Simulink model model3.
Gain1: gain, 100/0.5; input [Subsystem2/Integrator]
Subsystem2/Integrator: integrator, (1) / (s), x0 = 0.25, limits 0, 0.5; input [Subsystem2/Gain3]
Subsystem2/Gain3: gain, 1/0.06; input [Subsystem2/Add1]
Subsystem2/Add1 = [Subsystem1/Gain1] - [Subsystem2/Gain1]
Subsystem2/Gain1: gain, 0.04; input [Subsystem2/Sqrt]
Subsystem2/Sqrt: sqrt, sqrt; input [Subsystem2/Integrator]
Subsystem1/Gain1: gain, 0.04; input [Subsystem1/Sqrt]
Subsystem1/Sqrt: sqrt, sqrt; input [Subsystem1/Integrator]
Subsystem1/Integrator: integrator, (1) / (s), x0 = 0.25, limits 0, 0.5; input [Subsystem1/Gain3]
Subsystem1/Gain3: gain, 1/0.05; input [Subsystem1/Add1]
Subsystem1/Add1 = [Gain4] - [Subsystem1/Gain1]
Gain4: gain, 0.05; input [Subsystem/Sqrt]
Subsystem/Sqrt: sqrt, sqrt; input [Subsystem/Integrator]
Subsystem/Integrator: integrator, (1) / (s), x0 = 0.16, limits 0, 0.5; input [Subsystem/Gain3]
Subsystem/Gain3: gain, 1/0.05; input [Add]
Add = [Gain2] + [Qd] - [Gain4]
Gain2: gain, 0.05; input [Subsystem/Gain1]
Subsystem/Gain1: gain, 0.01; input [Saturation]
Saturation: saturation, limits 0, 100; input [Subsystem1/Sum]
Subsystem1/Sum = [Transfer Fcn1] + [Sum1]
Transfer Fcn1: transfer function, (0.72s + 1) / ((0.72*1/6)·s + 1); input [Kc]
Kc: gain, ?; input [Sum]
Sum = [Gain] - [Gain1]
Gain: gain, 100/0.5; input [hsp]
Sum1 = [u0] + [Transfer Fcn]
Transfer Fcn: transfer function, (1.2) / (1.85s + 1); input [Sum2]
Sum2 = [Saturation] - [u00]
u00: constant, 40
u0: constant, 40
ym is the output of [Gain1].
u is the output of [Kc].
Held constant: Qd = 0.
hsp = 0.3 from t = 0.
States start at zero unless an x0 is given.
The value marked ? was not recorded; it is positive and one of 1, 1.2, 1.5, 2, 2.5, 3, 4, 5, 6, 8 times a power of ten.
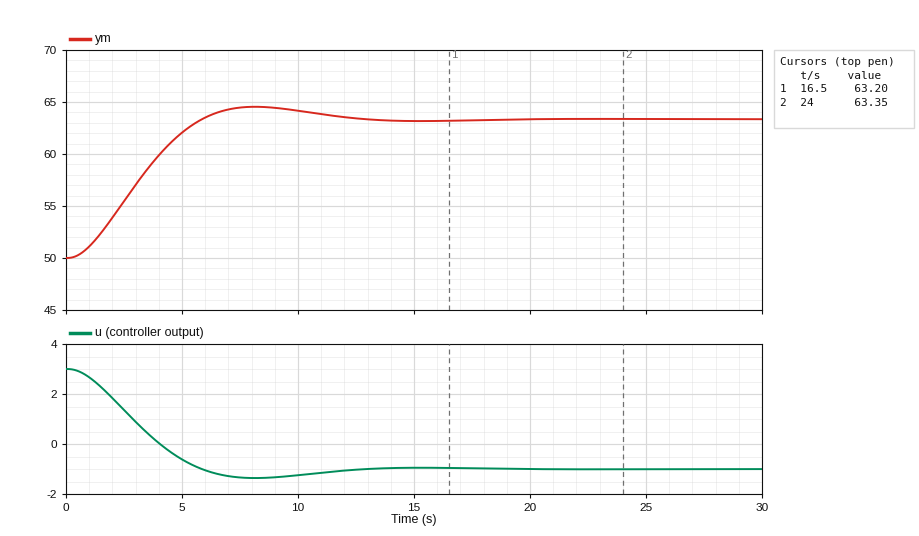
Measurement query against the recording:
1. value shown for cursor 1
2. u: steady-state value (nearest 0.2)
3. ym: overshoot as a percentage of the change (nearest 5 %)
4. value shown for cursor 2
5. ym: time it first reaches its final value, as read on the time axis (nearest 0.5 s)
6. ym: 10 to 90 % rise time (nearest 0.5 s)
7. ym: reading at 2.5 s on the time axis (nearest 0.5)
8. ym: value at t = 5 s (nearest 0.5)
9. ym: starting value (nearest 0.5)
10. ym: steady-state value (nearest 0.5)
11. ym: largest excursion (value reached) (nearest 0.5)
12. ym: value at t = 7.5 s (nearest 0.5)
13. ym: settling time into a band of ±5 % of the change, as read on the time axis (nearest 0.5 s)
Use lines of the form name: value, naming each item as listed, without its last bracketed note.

value shown for cursor 1: 63.20
u: steady-state value: -1.0
ym: overshoot as a percentage of the change: 10 %
value shown for cursor 2: 63.35
ym: time it first reaches its final value, as read on the time axis: 6.0 s
ym: 10 to 90 % rise time: 4.0 s
ym: reading at 2.5 s on the time axis: 55.5
ym: value at t = 5 s: 62.0
ym: starting value: 50.0
ym: steady-state value: 63.5
ym: largest excursion (value reached): 64.5
ym: value at t = 7.5 s: 64.5
ym: settling time into a band of ±5 % of the change, as read on the time axis: 10.5 s
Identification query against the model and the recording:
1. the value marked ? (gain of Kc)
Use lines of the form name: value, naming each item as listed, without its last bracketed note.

the value marked ?: 0.3
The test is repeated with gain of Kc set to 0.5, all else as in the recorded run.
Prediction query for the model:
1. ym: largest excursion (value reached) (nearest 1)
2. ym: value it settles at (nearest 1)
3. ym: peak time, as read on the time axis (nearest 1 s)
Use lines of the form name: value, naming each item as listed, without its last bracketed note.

ym: largest excursion (value reached): 65
ym: value it settles at: 62
ym: peak time, as read on the time axis: 5 s
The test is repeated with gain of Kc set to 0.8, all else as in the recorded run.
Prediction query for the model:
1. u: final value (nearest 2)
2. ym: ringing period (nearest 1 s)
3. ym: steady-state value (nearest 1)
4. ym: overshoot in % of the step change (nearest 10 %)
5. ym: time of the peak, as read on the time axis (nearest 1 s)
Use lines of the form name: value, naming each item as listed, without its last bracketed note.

u: final value: 0
ym: ringing period: 7 s
ym: steady-state value: 61
ym: overshoot in % of the step change: 40 %
ym: time of the peak, as read on the time axis: 4 s
